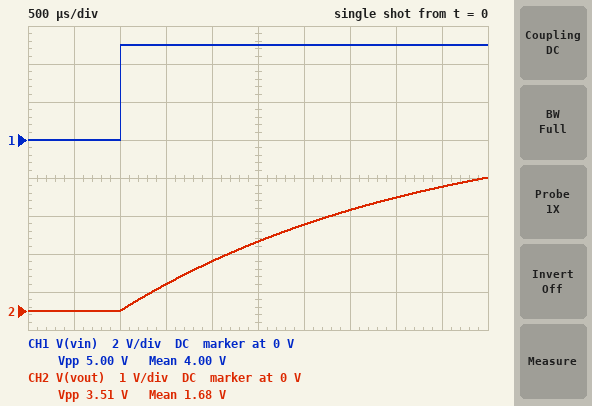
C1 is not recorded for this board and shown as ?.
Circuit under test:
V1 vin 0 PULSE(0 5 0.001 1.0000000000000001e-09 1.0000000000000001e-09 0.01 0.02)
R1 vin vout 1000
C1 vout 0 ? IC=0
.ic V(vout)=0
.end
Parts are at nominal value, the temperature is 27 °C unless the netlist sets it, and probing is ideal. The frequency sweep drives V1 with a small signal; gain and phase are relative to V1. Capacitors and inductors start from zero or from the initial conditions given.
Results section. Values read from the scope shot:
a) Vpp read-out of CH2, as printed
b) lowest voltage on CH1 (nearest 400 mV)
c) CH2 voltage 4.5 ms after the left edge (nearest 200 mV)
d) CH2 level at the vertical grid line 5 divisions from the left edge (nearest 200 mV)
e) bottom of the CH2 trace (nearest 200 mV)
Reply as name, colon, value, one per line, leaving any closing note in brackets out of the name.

Vpp read-out of CH2, as printed: 3.51 V
lowest voltage on CH1: 0 V
CH2 voltage 4.5 ms after the left edge: 3.2 V
CH2 level at the vertical grid line 5 divisions from the left edge: 1.8 V
bottom of the CH2 trace: 0 V
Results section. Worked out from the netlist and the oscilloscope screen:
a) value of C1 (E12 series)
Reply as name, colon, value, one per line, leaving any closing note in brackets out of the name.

value of C1: 3.3 µF
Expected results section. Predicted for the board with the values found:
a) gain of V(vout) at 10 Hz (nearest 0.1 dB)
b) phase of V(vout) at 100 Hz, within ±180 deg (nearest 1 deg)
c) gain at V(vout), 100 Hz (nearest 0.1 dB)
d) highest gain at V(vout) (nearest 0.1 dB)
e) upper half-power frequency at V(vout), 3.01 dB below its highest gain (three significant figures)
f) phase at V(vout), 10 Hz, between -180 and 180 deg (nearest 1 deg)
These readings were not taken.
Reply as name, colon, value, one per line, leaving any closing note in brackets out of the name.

gain of V(vout) at 10 Hz: -0.2 dB
phase of V(vout) at 100 Hz, within ±180 deg: -64 deg
gain at V(vout), 100 Hz: -7.2 dB
highest gain at V(vout): 0 dB
upper half-power frequency at V(vout), 3.01 dB below its highest gain: 48.2 Hz
phase at V(vout), 10 Hz, between -180 and 180 deg: -12 deg
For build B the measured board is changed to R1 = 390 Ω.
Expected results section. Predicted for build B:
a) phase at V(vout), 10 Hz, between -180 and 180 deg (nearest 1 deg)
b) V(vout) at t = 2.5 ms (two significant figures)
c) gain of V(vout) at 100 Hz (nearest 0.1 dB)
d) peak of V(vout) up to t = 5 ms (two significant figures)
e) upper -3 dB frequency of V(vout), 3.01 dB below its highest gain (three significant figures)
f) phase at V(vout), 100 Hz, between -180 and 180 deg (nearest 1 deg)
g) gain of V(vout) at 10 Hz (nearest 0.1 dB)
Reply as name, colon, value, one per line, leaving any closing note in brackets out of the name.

phase at V(vout), 10 Hz, between -180 and 180 deg: -5 deg
V(vout) at t = 2.5 ms: 3.4 V
gain of V(vout) at 100 Hz: -2.2 dB
peak of V(vout) up to t = 5 ms: 4.8 V
upper -3 dB frequency of V(vout), 3.01 dB below its highest gain: 124 Hz
phase at V(vout), 100 Hz, between -180 and 180 deg: -39 deg
gain of V(vout) at 10 Hz: 0 dB
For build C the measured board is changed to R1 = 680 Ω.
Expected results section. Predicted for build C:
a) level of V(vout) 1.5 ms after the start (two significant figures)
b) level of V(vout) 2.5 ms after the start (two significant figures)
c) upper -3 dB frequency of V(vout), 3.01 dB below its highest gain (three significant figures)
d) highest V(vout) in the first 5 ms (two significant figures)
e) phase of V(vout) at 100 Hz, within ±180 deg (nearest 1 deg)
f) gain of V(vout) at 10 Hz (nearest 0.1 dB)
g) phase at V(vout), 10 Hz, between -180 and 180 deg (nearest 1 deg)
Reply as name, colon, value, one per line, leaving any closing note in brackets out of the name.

level of V(vout) 1.5 ms after the start: 1.0 V
level of V(vout) 2.5 ms after the start: 2.4 V
upper -3 dB frequency of V(vout), 3.01 dB below its highest gain: 70.9 Hz
highest V(vout) in the first 5 ms: 4.2 V
phase of V(vout) at 100 Hz, within ±180 deg: -55 deg
gain of V(vout) at 10 Hz: -0.1 dB
phase at V(vout), 10 Hz, between -180 and 180 deg: -8 deg
